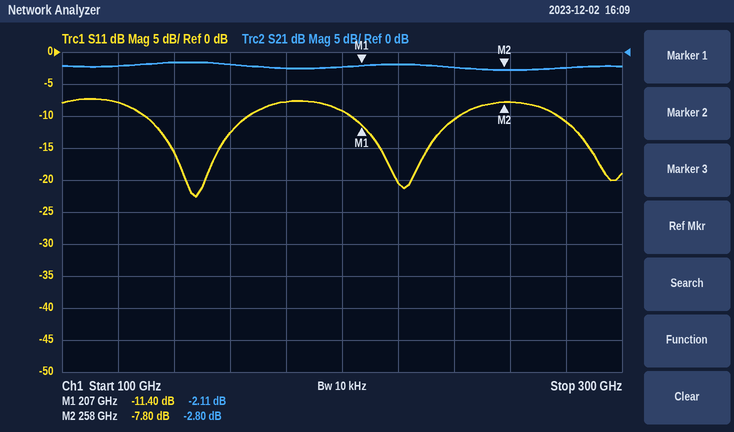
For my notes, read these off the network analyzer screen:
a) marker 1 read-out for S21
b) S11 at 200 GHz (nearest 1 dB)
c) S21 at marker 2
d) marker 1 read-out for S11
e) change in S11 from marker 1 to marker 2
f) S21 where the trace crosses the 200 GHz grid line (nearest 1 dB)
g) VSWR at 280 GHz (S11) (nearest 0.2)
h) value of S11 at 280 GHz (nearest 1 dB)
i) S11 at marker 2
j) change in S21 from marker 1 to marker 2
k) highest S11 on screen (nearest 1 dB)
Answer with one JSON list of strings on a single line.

["-2.11 dB", "-9 dB", "-2.80 dB", "-11.40 dB", "3.60 dB", "-2 dB", "1.8", "-11 dB", "-7.80 dB", "-0.69 dB", "-7 dB"]
